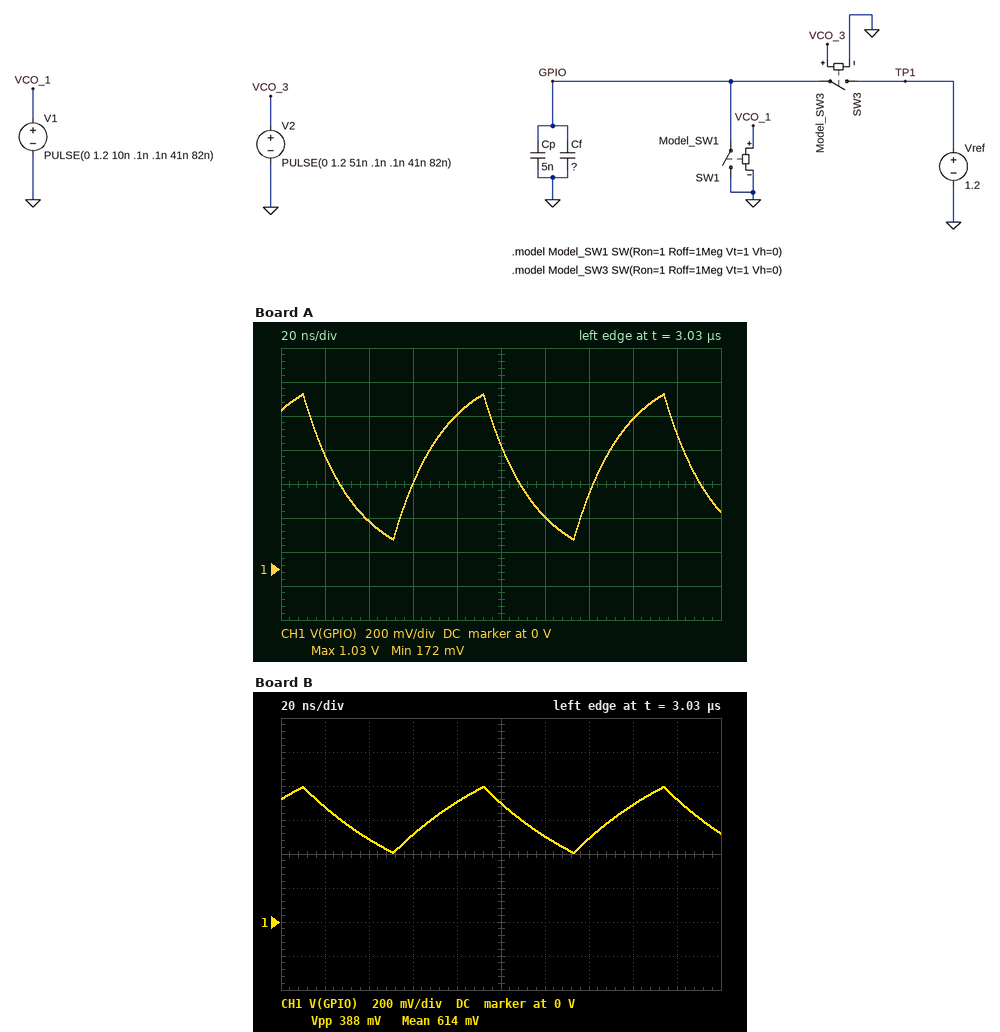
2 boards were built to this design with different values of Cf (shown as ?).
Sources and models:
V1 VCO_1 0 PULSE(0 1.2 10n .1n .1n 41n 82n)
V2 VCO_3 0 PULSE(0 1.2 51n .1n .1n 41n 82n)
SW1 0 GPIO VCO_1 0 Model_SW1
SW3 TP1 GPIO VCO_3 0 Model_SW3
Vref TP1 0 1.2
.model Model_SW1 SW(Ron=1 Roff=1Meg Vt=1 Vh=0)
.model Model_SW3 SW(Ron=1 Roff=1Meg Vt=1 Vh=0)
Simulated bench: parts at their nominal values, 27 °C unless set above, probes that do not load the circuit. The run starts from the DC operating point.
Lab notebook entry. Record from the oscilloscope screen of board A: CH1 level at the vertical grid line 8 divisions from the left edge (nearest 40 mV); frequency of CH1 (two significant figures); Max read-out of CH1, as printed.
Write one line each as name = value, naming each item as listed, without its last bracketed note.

CH1 level at the vertical grid line 8 divisions from the left edge = 880 mV
frequency of CH1 = 12 MHz
Max read-out of CH1, as printed = 1.03 V
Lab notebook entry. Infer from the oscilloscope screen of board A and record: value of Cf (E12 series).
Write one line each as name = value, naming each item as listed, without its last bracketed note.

value of Cf = 18 nF
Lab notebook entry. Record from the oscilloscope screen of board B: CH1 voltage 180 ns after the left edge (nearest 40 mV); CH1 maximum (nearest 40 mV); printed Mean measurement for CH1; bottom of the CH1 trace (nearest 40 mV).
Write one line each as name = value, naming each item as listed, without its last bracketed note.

CH1 voltage 180 ns after the left edge = 720 mV
CH1 maximum = 800 mV
printed Mean measurement for CH1 = 614 mV
bottom of the CH1 trace = 400 mV
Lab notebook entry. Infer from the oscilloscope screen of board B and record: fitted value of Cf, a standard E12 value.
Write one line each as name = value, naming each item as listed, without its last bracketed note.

fitted value of Cf, a standard E12 value = 56 nF
